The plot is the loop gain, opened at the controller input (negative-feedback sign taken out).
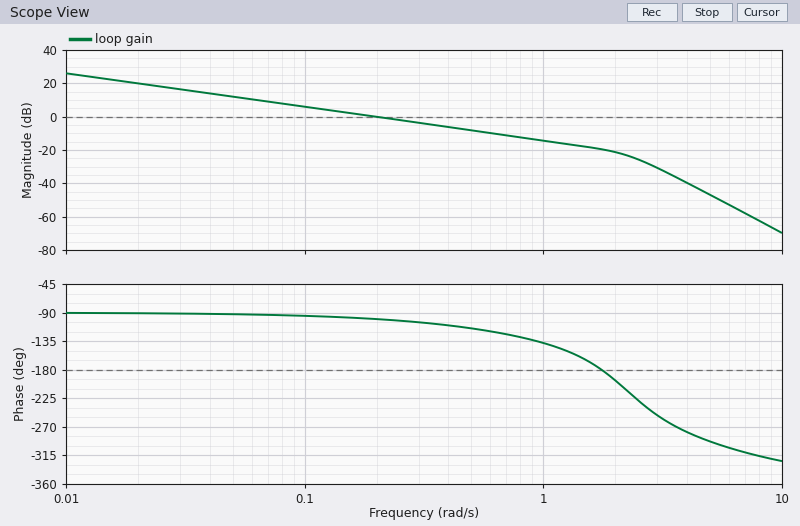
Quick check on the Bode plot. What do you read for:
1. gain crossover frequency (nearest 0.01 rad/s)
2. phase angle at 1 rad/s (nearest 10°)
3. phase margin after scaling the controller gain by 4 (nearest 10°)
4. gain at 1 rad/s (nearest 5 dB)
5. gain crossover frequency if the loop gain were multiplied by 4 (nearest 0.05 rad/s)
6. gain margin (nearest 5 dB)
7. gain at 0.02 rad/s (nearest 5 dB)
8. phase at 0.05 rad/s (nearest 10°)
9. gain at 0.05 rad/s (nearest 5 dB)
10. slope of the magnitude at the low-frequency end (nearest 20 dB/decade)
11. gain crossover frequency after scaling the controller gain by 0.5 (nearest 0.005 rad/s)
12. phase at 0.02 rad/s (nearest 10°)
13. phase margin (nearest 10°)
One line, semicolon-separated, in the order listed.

0.20 rad/s; -140°; 50°; -15 dB; 0.75 rad/s; 20 dB; 20 dB; -90°; 10 dB; -20 dB/decade; 0.100 rad/s; -90°; 80°
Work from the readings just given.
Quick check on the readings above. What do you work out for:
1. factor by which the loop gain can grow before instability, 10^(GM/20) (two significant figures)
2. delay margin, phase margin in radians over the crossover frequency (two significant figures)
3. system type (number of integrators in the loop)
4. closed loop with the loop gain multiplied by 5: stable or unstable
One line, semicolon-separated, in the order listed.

10; 7.0 s; 1; stable
